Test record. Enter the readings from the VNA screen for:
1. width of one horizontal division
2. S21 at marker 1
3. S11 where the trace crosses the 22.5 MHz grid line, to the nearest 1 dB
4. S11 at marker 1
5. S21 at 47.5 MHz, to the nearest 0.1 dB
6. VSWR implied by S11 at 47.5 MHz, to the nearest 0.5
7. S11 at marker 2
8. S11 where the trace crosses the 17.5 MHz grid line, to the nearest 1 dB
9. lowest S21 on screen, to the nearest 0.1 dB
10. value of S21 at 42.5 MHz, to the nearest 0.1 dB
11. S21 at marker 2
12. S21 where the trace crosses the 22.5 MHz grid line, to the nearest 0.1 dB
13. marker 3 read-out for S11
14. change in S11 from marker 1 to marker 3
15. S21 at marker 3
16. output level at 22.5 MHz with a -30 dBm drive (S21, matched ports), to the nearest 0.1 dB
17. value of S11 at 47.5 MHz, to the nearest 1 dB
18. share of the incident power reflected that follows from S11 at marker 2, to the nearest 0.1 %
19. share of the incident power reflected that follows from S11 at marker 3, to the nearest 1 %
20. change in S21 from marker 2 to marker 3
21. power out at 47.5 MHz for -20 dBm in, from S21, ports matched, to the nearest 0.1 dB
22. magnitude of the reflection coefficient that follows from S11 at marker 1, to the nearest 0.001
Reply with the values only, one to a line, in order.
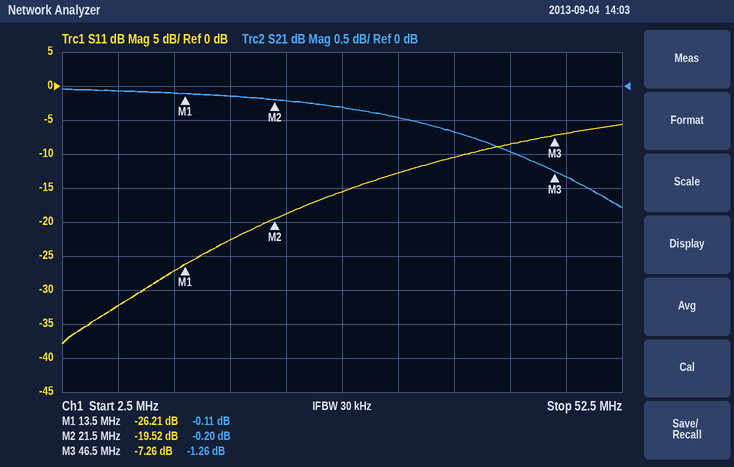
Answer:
5 MHz
-0.11 dB
-19 dB
-26.21 dB
-1.3 dB
2.5
-19.52 dB
-23 dB
-1.8 dB
-1.0 dB
-0.20 dB
-0.2 dB
-7.26 dB
18.95 dB
-1.26 dB
-30.2 dBm
-7 dB
1.1 %
19 %
-1.06 dB
-21.3 dBm
0.049
